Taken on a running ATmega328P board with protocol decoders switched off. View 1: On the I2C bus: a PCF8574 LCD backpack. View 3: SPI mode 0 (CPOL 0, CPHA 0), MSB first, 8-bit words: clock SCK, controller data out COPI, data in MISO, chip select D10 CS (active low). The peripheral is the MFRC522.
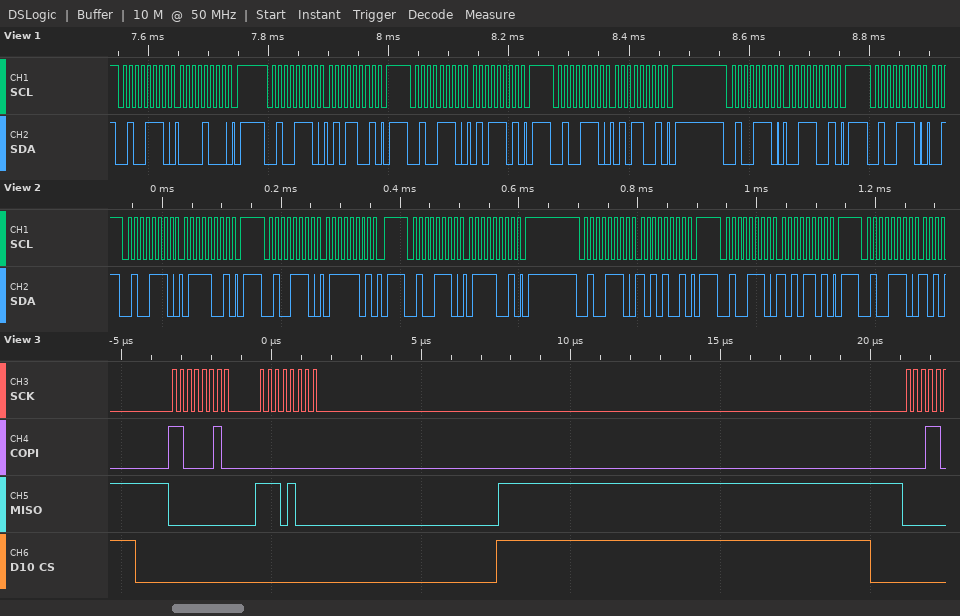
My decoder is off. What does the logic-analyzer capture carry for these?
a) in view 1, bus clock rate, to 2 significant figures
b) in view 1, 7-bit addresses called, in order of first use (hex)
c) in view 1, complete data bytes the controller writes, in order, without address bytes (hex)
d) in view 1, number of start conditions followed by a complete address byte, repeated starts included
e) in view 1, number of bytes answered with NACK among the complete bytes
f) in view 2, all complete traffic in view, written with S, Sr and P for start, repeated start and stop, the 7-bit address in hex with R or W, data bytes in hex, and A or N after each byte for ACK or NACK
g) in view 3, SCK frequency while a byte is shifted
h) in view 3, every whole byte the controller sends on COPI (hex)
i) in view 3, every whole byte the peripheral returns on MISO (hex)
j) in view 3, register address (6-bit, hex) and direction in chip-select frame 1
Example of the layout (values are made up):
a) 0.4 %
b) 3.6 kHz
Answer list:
a) 100 kHz
b) 0x27
c) 08 59 5D 59 39
d) 6
e) 0
f) S 27W A 79 A P S 27W A 7D A P S 27W A 79 A P S 27W A A9 A P S 27W A AD A P S 27W A
g) 4 MHz
h) C2 00
i) 00 E8
j) 0x21 read
